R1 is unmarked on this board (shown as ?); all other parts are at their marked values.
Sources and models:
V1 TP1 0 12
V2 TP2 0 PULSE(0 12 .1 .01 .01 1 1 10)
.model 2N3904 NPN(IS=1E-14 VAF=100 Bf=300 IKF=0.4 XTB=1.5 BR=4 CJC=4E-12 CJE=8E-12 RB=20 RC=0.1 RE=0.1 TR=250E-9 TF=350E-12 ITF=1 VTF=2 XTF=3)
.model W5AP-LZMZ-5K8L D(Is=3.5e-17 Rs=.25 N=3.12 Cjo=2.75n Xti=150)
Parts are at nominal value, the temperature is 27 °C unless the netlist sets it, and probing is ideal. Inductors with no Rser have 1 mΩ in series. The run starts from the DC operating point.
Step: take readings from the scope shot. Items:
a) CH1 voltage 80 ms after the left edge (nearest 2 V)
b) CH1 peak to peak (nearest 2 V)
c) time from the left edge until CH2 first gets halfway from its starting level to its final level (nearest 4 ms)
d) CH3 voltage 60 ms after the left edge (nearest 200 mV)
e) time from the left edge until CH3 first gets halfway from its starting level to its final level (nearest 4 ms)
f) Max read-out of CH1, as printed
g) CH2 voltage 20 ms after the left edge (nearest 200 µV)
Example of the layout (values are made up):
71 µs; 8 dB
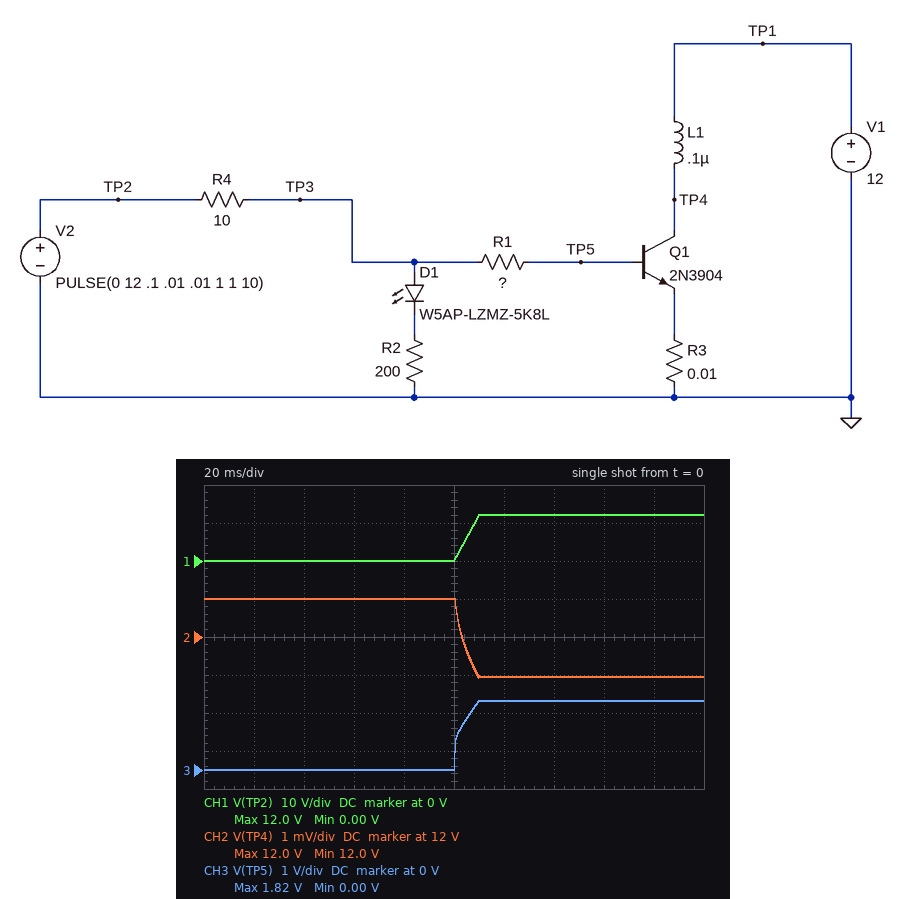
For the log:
0 V; 12 V; 104 ms; 0 V; 100 ms; 12.0 V; 12.0000 V
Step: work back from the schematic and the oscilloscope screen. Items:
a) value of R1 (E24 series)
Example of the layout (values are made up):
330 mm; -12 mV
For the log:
270 Ω
